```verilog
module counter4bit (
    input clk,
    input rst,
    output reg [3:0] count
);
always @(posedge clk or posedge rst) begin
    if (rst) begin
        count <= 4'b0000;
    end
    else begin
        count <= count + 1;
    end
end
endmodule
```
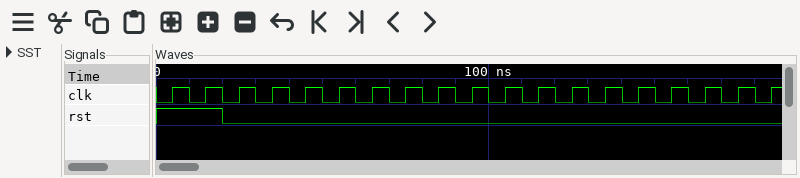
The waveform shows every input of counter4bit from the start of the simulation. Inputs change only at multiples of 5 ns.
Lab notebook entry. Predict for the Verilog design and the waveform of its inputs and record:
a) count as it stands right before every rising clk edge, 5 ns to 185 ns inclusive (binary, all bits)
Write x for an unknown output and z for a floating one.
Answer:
0000, 0000, 0000, 0001, 0010, 0011, 0100, 0101, 0110, 0111, 1000, 1001, 1010, 1011, 1100, 1101, 1110, 1111, 0000
